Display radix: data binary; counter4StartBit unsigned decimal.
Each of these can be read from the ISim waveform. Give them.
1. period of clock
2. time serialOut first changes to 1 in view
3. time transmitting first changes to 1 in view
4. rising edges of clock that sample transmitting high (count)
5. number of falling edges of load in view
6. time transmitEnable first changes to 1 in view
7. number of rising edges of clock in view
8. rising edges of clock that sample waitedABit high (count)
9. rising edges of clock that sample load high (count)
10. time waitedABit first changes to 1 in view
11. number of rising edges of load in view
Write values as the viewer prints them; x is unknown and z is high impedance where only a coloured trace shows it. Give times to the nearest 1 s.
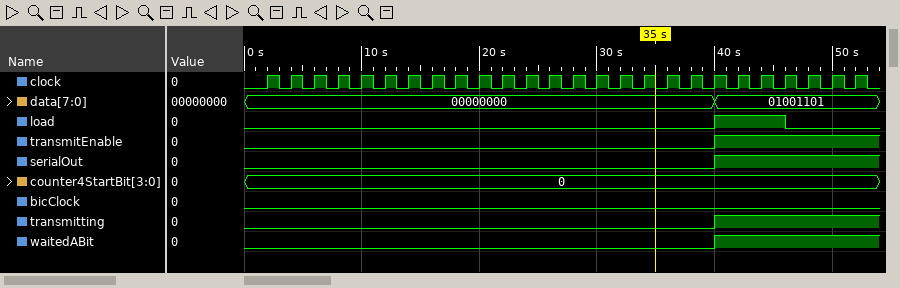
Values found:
2 s
40 s
40 s
6
1
40 s
26
6
3
40 s
1
